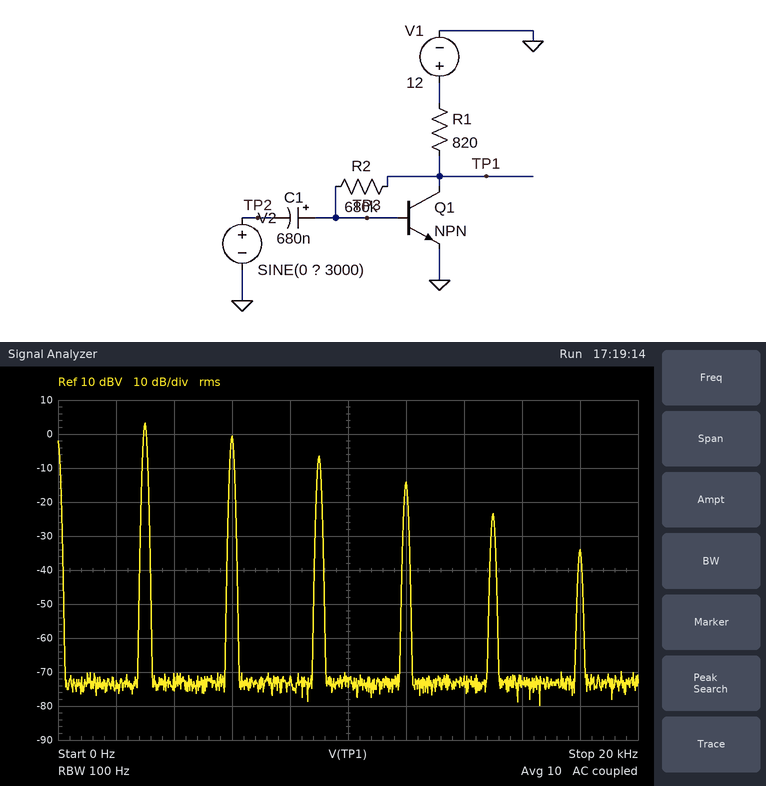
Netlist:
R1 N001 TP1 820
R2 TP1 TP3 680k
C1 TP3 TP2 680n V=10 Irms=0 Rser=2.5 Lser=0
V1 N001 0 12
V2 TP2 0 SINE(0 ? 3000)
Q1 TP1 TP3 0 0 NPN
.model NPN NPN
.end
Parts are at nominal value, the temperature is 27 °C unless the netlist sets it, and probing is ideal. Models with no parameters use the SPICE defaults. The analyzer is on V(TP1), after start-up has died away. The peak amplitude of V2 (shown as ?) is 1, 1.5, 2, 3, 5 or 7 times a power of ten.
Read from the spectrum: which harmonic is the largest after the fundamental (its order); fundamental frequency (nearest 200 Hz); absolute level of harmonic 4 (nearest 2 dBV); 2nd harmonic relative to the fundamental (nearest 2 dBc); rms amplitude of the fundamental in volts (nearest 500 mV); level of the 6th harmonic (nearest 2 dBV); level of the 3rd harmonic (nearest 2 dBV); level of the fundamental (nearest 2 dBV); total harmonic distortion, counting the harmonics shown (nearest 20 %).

2
3.0 kHz
-14 dBV
-4 dBc
1.5 V
-34 dBV
-6 dBV
4 dBV
80 %
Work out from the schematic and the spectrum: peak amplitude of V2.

100 mV
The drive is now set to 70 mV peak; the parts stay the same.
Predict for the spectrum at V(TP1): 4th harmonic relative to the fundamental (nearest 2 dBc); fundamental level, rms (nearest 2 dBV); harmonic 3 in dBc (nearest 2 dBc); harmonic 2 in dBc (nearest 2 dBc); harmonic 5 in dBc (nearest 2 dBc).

-24 dBc
2 dBV
-14 dBc
-6 dBc
-36 dBc
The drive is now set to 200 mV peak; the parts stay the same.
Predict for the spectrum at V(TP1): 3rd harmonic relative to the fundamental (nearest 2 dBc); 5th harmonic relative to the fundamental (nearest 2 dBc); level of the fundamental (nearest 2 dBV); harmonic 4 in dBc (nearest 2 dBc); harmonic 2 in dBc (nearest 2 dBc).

-4 dBc
-14 dBc
4 dBV
-8 dBc
-2 dBc
